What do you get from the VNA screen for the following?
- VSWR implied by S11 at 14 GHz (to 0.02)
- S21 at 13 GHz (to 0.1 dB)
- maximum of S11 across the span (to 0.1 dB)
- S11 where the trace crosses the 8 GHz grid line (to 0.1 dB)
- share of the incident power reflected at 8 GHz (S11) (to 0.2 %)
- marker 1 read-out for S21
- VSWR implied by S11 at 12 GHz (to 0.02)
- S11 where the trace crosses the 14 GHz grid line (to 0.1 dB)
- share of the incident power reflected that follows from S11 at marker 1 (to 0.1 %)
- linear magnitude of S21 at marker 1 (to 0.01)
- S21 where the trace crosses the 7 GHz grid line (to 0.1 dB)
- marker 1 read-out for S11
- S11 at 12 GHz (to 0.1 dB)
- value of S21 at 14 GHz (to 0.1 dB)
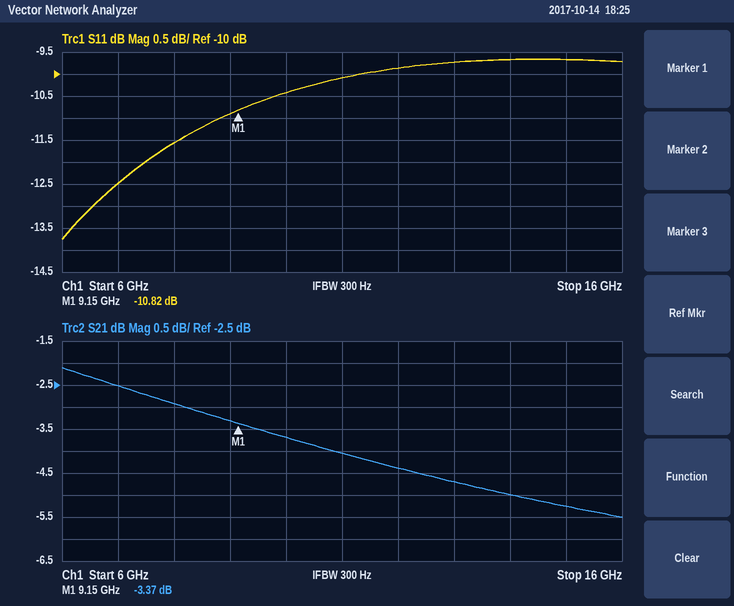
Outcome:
1.98
-4.7 dB
-9.7 dB
-11.6 dB
7.0 %
-3.37 dB
1.94
-9.7 dB
8.3 %
0.68
-2.5 dB
-10.82 dB
-9.9 dB
-5.0 dB
